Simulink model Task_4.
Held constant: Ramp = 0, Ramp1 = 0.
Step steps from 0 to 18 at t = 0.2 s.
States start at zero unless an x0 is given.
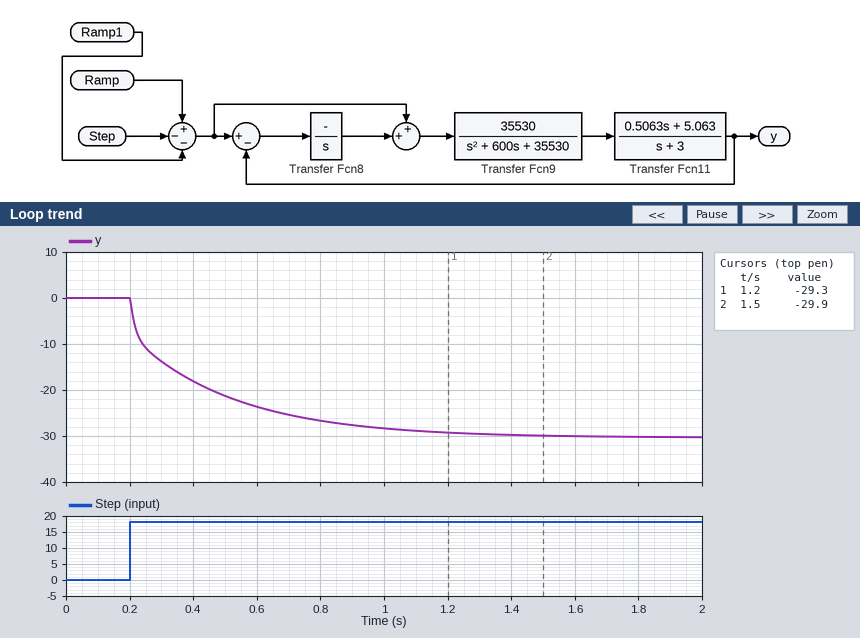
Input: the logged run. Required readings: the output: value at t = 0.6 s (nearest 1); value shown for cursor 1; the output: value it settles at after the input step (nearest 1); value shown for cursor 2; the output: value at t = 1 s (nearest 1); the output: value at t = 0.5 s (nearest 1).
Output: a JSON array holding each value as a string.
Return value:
["-24", "-29.3", "-30", "-29.9", "-28", "-21"]
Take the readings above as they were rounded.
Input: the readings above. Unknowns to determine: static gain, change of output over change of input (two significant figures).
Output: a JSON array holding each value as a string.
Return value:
["-1.7"]
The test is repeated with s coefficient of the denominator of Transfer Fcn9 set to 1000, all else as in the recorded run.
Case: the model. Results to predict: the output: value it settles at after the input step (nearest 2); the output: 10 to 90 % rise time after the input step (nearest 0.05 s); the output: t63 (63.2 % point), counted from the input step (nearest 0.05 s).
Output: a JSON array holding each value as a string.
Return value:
["-30", "0.65 s", "0.25 s"]
